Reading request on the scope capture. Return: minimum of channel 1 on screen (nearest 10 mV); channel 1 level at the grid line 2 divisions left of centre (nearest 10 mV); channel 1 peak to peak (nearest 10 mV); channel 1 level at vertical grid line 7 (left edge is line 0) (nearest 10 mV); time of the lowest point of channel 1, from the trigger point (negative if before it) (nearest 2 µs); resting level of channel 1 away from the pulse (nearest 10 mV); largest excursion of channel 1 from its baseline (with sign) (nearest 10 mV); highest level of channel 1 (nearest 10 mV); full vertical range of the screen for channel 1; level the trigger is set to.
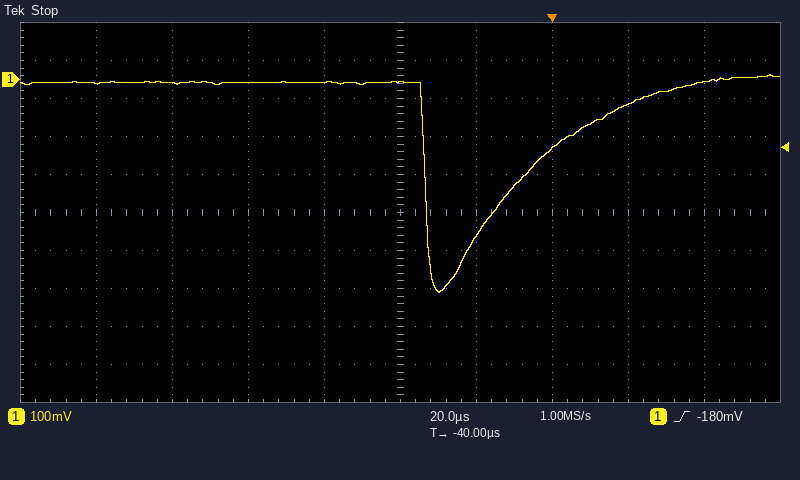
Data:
-560 mV
-10 mV
570 mV
-180 mV
-30 µs
-10 mV
-550 mV
10 mV
1 V
-180 mV
